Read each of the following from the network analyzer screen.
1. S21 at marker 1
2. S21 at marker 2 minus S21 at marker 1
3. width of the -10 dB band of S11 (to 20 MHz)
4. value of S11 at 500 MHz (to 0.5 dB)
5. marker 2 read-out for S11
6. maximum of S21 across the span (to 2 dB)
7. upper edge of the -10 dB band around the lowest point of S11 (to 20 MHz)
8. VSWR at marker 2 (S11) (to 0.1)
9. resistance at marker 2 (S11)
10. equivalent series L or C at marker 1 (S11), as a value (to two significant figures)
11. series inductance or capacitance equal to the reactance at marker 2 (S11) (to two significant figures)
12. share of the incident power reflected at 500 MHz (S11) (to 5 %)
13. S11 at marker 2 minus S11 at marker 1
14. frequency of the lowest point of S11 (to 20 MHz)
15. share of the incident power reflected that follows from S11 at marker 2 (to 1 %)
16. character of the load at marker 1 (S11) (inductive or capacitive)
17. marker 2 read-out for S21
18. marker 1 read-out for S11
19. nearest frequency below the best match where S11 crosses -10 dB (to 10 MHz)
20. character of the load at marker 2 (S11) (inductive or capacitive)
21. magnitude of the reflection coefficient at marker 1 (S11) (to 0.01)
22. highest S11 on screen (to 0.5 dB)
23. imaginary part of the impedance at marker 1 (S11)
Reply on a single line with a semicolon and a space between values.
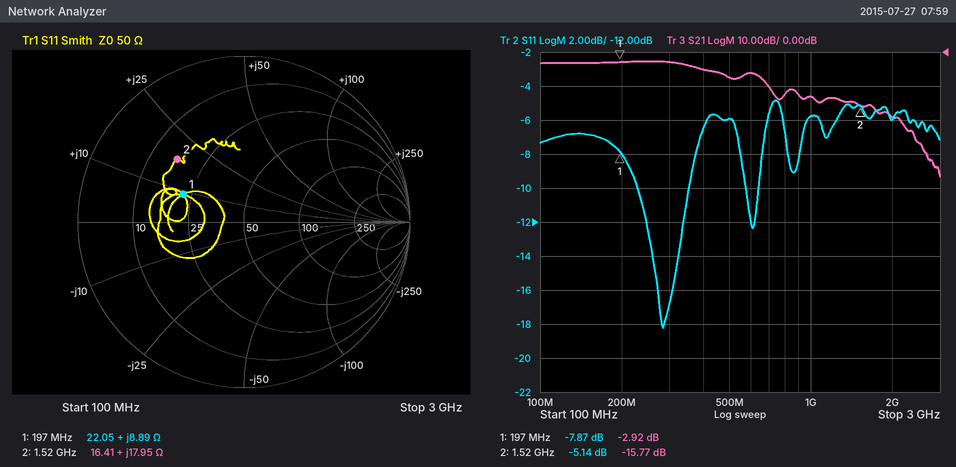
-2.92 dB; -12.85 dB; 120 MHz; -6.0 dB; -5.14 dB; -2 dB; 360 MHz; 3.5; 16.41 Ω; 7.2 nH; 1.9 nH; 25 %; 2.73 dB; 280 MHz; 31 %; inductive; -15.77 dB; -7.87 dB; 230 MHz; inductive; 0.40; -5.0 dB; +8.89 Ω
